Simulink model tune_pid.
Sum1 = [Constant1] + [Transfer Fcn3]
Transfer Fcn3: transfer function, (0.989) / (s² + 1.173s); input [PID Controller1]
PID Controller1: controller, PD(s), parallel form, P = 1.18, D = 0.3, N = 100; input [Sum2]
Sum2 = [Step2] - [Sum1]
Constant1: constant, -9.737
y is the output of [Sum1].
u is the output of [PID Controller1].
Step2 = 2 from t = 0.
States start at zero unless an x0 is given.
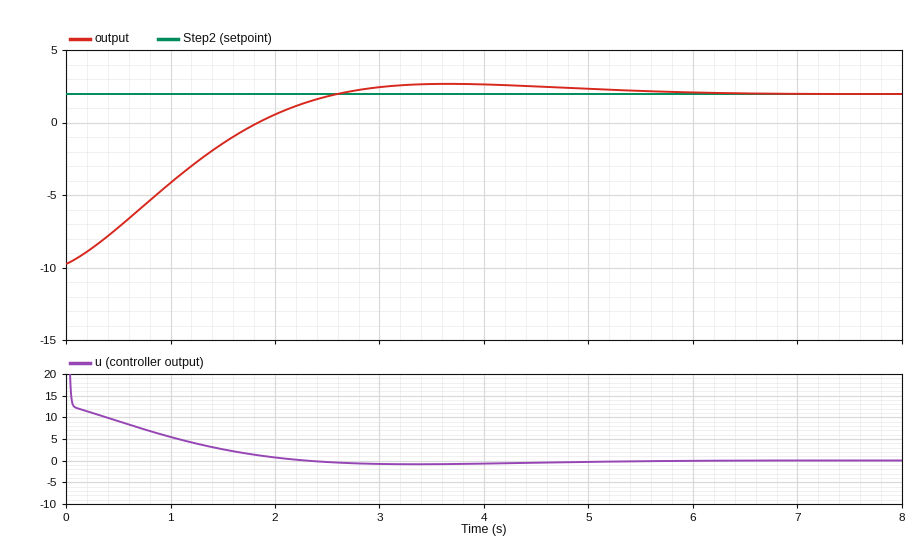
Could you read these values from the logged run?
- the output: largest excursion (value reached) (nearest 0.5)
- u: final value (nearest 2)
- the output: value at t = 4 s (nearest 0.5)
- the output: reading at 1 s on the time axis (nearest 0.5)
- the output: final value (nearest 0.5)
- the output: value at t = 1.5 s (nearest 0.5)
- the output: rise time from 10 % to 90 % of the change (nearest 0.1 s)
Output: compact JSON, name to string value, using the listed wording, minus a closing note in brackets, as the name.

{"the output: largest excursion (value reached)": "2.5", "u: final value": "0", "the output: value at t = 4 s": "2.5", "the output: reading at 1 s on the time axis": "-4.0", "the output: final value": "2.0", "the output: value at t = 1.5 s": "-1.5", "the output: rise time from 10 % to 90 % of the change": "1.8 s"}
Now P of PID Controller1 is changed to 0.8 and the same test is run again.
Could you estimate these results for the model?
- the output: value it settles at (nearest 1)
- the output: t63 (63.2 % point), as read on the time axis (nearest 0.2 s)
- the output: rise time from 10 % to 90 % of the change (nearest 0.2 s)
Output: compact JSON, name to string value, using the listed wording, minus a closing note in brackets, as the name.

{"the output: value it settles at": "2", "the output: t63 (63.2 % point), as read on the time axis": "1.8 s", "the output: rise time from 10 % to 90 % of the change": "2.8 s"}
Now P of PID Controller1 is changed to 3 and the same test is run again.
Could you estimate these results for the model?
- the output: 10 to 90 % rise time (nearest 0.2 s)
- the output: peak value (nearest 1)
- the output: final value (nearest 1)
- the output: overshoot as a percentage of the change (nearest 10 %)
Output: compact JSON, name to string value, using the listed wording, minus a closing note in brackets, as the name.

{"the output: 10 to 90 % rise time": "0.8 s", "the output: peak value": "5", "the output: final value": "2", "the output: overshoot as a percentage of the change": "20 %"}
